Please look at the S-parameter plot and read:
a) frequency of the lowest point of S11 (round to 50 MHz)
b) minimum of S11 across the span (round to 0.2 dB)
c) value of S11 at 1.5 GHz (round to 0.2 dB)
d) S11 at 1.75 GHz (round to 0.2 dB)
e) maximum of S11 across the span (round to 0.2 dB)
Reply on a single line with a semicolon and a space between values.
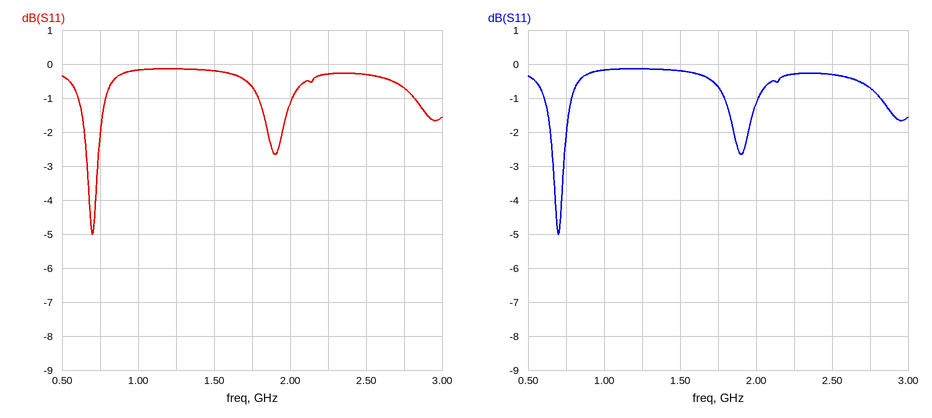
700 MHz; -5.0 dB; -0.2 dB; -0.6 dB; -0.2 dB
